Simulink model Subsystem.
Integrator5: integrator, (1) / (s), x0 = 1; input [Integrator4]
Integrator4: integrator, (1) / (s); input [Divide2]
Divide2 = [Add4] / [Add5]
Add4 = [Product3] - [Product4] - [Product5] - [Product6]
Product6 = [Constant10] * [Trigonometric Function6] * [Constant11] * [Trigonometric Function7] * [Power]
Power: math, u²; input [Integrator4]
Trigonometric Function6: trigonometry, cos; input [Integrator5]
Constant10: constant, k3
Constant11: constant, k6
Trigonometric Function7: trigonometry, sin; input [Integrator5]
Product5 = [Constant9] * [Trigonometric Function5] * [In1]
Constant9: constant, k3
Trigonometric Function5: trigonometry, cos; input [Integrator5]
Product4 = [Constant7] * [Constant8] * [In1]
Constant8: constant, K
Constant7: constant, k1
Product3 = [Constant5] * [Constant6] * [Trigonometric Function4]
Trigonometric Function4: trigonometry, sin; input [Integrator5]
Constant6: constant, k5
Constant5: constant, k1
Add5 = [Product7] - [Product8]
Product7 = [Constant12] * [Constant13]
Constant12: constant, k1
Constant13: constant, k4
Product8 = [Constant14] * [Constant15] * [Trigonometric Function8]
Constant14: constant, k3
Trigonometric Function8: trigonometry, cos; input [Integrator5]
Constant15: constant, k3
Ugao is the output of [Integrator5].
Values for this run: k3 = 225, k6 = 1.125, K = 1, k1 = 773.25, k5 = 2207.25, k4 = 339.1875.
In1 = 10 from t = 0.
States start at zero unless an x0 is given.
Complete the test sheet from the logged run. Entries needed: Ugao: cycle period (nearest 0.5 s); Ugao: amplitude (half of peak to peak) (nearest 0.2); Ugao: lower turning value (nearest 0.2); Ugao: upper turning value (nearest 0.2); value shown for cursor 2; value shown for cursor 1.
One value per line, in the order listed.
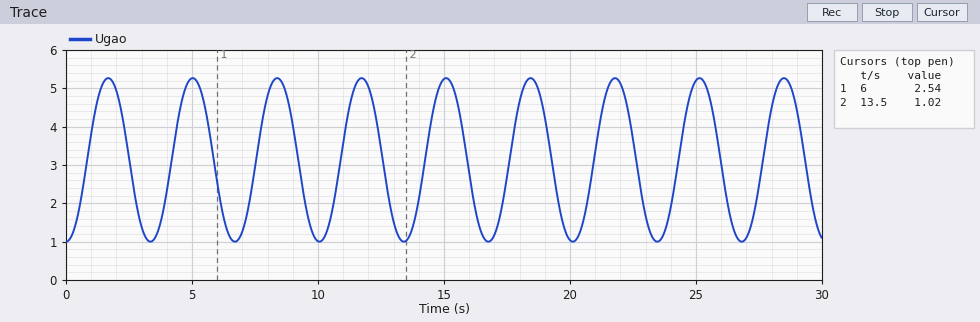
3.5 s
2.2
1.0
5.2
1.02
2.54
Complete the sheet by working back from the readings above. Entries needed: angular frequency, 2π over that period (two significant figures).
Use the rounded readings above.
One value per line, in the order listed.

1.8 rad/s
